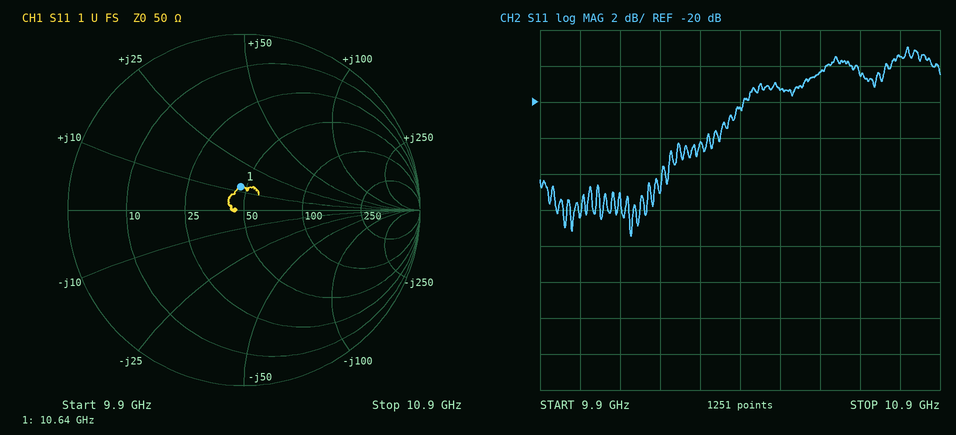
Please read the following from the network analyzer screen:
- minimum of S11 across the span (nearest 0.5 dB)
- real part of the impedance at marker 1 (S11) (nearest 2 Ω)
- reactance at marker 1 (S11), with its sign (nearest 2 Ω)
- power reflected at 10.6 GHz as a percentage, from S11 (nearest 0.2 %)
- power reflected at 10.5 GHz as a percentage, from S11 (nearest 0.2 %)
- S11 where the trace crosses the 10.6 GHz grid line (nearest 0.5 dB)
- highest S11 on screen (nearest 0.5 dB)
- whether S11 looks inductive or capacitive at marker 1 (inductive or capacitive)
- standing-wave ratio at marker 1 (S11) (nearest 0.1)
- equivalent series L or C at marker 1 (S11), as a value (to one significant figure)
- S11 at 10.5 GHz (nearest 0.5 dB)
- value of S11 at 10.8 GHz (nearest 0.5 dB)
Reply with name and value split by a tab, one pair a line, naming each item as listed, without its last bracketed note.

minimum of S11 across the span	-27.5 dB
real part of the impedance at marker 1 (S11)	46 Ω
reactance at marker 1 (S11), with its sign	+12 Ω
power reflected at 10.6 GHz as a percentage, from S11	1.4 %
power reflected at 10.5 GHz as a percentage, from S11	1.2 %
S11 where the trace crosses the 10.6 GHz grid line	-18.5 dB
highest S11 on screen	-17.0 dB
whether S11 looks inductive or capacitive at marker 1	inductive
standing-wave ratio at marker 1 (S11)	1.3
equivalent series L or C at marker 1 (S11), as a value	200 pH
S11 at 10.5 GHz	-19.5 dB
value of S11 at 10.8 GHz	-17.5 dB
